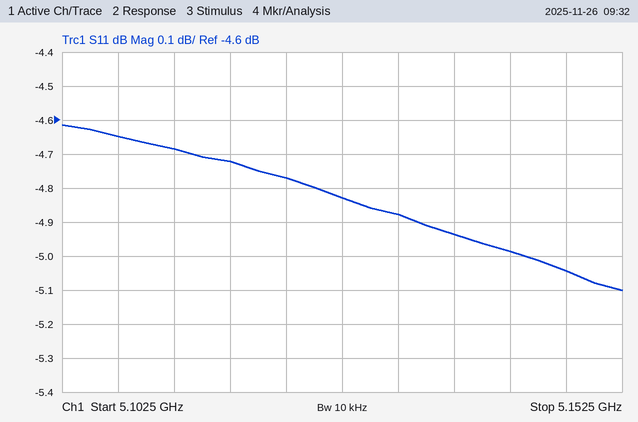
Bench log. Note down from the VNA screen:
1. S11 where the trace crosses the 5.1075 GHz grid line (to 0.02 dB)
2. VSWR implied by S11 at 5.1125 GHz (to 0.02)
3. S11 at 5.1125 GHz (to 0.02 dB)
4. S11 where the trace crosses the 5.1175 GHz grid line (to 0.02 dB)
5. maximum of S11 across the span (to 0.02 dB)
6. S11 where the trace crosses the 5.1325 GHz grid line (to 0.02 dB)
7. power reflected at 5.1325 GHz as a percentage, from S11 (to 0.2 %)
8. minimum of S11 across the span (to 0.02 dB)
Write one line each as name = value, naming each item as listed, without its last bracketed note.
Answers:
S11 where the trace crosses the 5.1075 GHz grid line = -4.64 dB
VSWR implied by S11 at 5.1125 GHz = 3.80
S11 at 5.1125 GHz = -4.68 dB
S11 where the trace crosses the 5.1175 GHz grid line = -4.72 dB
maximum of S11 across the span = -4.62 dB
S11 where the trace crosses the 5.1325 GHz grid line = -4.88 dB
power reflected at 5.1325 GHz as a percentage, from S11 = 32.6 %
minimum of S11 across the span = -5.10 dB
